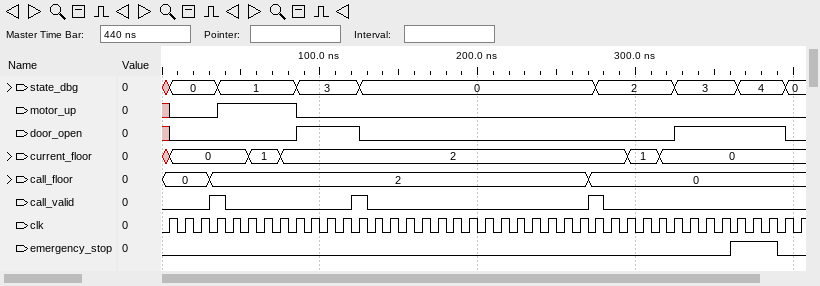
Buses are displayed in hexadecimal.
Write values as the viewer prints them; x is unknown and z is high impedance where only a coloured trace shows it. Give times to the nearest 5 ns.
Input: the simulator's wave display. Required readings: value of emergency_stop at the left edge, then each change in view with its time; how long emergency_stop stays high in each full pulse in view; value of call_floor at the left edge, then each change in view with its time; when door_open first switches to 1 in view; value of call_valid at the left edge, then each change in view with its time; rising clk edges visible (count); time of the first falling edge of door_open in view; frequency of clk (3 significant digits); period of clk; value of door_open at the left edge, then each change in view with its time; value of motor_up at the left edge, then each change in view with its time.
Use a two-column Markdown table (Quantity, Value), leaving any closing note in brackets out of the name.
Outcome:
| Quantity | Value |
|---|---|
| value of emergency_stop at the left edge, then each change in view with its time | 0, 1 at 360 ns, 0 at 390 ns |
| how long emergency_stop stays high in each full pulse in view | 30 ns |
| value of call_floor at the left edge, then each change in view with its time | 0, 2 at 30 ns, 0 at 270 ns |
| when door_open first switches to 1 in view | 85 ns |
| value of call_valid at the left edge, then each change in view with its time | 0, 1 at 30 ns, 0 at 40 ns, 1 at 120 ns, 0 at 130 ns, 1 at 270 ns, 0 at 280 ns |
| rising clk edges visible | 41 |
| time of the first falling edge of door_open in view | 125 ns |
| frequency of clk | 100 MHz |
| period of clk | 10 ns |
| value of door_open at the left edge, then each change in view with its time | x, 0 at 5 ns, 1 at 85 ns, 0 at 125 ns, 1 at 325 ns, 0 at 395 ns |
| value of motor_up at the left edge, then each change in view with its time | x, 0 at 5 ns, 1 at 35 ns, 0 at 85 ns |
